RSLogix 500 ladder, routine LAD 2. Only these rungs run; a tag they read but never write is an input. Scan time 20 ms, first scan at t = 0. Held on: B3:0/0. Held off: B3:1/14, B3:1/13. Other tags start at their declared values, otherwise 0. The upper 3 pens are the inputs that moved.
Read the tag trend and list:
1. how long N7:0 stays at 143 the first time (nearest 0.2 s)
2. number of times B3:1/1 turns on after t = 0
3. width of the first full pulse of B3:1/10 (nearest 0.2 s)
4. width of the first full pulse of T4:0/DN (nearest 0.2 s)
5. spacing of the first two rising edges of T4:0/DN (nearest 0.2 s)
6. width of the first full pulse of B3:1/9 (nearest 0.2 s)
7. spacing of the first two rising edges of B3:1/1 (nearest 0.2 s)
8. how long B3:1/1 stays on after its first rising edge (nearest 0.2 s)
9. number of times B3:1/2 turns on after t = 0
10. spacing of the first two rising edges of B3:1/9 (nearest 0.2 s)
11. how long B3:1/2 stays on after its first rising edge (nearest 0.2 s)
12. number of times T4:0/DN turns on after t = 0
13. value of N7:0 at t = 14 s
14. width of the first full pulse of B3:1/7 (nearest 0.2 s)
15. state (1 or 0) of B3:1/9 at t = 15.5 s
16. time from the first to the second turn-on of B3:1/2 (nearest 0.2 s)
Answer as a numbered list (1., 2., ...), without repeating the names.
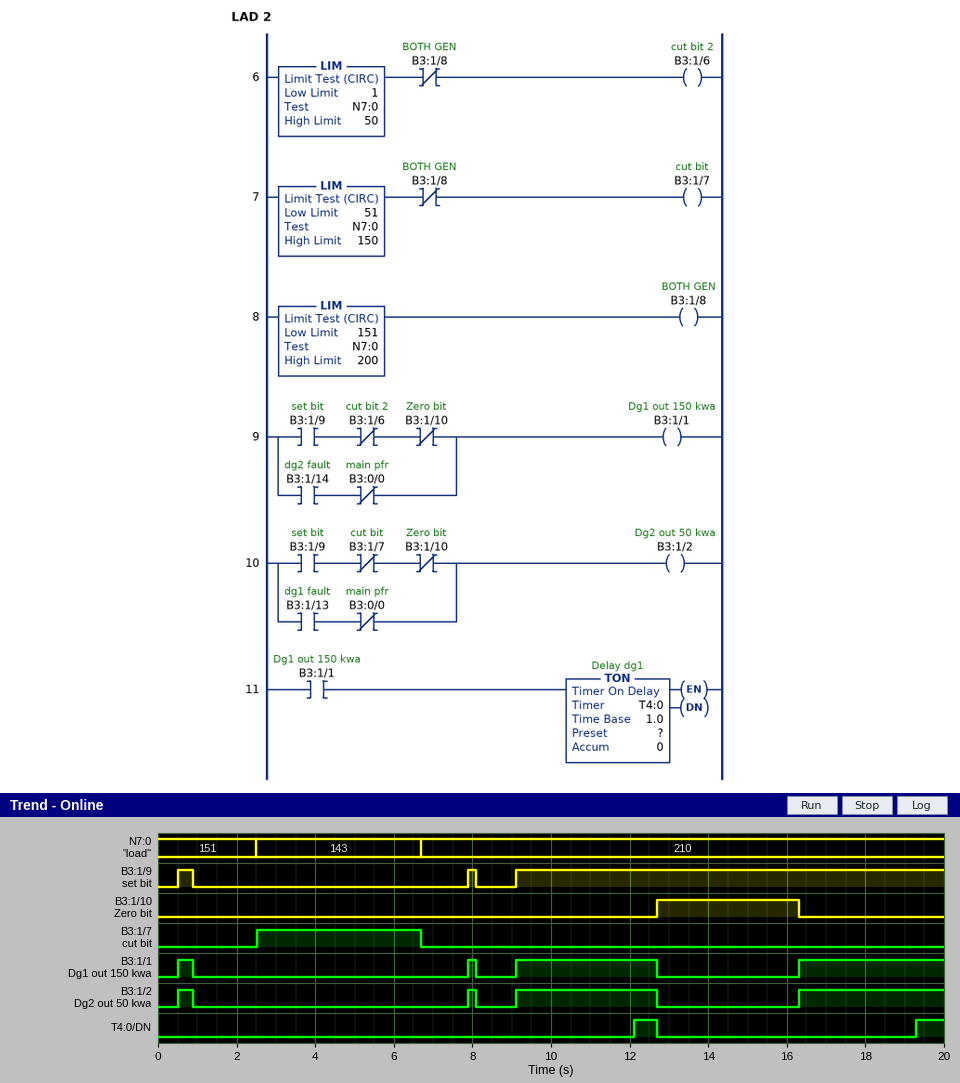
1. 4.2 s
2. 4
3. 3.6 s
4. 0.6 s
5. 7.2 s
6. 0.4 s
7. 7.4 s
8. 0.4 s
9. 4
10. 7.4 s
11. 0.4 s
12. 2
13. 210
14. 4.2 s
15. 1
16. 7.4 s
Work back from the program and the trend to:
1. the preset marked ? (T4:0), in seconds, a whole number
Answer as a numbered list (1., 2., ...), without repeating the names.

1. 3 s
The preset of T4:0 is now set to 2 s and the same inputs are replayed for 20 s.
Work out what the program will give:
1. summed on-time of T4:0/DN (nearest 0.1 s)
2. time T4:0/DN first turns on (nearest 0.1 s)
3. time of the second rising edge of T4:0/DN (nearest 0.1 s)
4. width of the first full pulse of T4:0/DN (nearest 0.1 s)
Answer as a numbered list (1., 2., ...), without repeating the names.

1. 3.3 s
2. 11.1 s
3. 18.3 s
4. 1.6 s
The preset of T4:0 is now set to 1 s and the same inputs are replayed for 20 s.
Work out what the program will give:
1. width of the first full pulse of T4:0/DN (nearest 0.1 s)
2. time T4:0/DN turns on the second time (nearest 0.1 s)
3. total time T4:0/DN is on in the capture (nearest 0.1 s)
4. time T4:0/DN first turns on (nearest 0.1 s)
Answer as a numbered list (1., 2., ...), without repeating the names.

1. 2.6 s
2. 17.3 s
3. 5.3 s
4. 10.1 s
